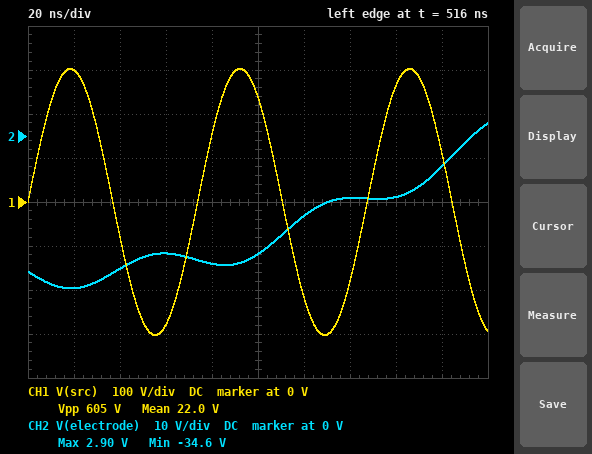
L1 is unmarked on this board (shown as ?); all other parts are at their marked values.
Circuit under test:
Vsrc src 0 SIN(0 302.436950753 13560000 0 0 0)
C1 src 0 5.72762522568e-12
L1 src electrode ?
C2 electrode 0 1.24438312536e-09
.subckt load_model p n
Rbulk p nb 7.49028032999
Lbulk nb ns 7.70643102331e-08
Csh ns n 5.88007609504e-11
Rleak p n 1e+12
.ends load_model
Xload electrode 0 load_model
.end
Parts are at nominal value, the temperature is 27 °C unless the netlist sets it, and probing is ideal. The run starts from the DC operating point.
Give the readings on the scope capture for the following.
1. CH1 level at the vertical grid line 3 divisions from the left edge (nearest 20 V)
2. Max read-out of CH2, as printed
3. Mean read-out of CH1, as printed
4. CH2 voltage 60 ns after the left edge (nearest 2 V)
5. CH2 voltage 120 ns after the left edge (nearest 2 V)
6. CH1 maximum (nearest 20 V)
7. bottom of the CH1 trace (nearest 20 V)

-280 V
2.90 V
22.0 V
-26 V
-18 V
300 V
-300 V
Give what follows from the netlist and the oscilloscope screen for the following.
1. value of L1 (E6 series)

10 µH
